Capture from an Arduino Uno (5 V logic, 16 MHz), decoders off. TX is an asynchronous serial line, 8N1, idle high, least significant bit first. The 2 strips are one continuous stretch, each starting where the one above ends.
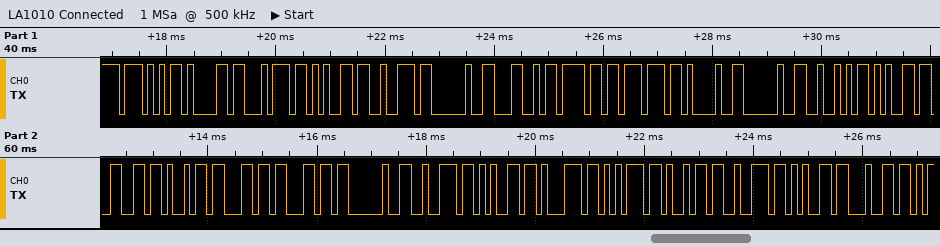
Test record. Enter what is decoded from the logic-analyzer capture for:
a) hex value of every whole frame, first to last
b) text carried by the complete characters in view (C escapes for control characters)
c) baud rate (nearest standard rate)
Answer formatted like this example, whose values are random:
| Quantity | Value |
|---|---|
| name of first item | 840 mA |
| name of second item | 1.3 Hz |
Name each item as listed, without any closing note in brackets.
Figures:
| Quantity | Value |
|---|---|
| hex value of every whole frame, first to last | 57 61 74 65 72 20 4C 6F 77 21 20 52 65 66 69 6C 6C 20 72 65 71 75 69 72 65 64 |
| text carried by the complete characters in view | "Water Low! Refill required" |
| baud rate | 9600 baud |
